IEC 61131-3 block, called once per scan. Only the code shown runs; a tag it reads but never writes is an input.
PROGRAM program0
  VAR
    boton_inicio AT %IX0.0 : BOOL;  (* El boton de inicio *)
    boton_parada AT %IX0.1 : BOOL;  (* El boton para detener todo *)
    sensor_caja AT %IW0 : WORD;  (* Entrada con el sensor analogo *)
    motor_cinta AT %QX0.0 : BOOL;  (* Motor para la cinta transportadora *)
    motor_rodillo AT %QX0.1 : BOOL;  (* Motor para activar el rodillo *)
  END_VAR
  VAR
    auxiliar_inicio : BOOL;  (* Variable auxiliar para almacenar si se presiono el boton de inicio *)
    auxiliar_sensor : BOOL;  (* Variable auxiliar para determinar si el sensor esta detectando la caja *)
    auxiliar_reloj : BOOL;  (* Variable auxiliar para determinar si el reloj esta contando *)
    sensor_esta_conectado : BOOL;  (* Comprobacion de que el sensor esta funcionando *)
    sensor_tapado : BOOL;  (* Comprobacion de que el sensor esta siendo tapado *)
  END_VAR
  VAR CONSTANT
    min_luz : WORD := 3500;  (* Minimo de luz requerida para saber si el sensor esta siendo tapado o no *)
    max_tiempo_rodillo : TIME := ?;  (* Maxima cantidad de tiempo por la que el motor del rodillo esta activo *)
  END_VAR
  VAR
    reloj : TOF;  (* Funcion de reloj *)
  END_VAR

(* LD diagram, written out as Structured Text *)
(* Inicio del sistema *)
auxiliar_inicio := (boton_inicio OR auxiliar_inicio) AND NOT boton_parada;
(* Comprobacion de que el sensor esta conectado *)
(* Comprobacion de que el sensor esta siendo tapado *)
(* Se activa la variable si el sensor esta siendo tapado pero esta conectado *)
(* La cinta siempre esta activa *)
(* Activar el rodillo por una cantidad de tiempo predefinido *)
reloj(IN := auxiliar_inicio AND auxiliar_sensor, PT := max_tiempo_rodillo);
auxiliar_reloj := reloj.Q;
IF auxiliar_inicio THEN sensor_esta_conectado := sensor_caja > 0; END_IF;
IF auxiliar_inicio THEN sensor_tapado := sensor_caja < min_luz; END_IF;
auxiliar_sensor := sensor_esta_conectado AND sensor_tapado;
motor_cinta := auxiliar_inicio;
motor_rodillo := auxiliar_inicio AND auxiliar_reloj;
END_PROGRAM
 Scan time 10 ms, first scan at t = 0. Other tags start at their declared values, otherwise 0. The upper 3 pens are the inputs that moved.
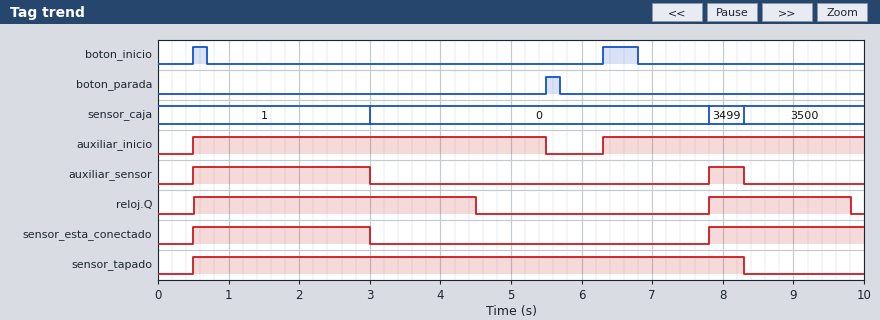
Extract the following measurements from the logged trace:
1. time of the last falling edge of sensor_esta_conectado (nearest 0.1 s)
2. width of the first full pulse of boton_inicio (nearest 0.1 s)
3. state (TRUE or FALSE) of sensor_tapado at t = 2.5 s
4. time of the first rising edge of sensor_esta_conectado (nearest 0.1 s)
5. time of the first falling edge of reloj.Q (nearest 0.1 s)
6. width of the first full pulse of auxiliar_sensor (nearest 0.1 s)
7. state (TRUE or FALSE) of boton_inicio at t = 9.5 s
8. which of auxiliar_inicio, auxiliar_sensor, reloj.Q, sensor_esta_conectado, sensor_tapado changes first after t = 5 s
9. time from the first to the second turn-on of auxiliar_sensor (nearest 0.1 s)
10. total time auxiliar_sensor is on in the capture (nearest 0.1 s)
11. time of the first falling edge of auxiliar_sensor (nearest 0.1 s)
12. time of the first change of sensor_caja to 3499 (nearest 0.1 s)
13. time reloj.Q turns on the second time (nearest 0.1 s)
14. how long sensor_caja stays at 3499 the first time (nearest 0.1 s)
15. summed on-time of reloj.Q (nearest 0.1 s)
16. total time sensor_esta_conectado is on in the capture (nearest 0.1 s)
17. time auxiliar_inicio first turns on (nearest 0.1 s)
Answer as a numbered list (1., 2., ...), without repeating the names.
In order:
1. 3.0 s
2. 0.2 s
3. TRUE
4. 0.5 s
5. 4.5 s
6. 2.5 s
7. FALSE
8. auxiliar_inicio
9. 7.3 s
10. 3.0 s
11. 3.0 s
12. 7.8 s
13. 7.8 s
14. 0.5 s
15. 6.0 s
16. 4.7 s
17. 0.5 s
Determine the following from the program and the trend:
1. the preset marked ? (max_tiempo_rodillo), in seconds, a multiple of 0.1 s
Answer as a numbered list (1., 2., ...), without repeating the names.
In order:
1. 1.5 s
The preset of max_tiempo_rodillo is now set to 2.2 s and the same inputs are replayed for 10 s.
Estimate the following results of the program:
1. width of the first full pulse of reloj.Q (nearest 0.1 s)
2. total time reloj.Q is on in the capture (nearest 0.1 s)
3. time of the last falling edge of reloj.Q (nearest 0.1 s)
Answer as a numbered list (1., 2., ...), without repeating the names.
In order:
1. 4.7 s
2. 6.9 s
3. 5.2 s
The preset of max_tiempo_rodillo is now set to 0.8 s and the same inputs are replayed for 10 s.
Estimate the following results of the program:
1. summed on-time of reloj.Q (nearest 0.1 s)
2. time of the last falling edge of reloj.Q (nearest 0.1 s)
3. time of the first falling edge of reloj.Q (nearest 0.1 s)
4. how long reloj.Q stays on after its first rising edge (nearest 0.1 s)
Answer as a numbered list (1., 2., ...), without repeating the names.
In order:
1. 4.6 s
2. 9.1 s
3. 3.8 s
4. 3.3 s
